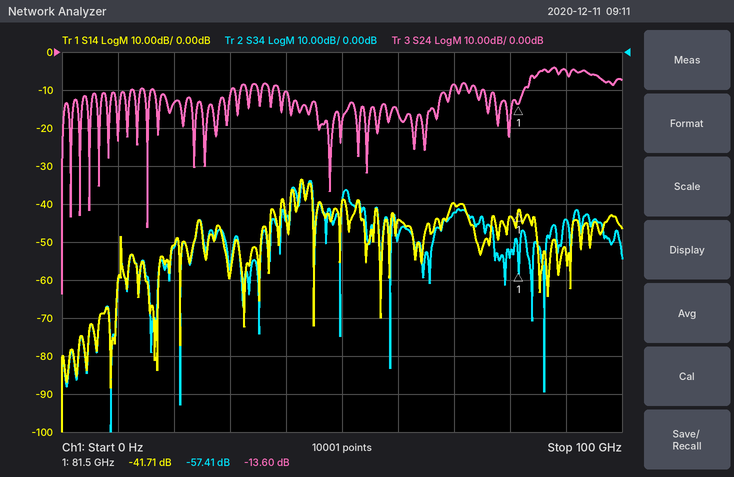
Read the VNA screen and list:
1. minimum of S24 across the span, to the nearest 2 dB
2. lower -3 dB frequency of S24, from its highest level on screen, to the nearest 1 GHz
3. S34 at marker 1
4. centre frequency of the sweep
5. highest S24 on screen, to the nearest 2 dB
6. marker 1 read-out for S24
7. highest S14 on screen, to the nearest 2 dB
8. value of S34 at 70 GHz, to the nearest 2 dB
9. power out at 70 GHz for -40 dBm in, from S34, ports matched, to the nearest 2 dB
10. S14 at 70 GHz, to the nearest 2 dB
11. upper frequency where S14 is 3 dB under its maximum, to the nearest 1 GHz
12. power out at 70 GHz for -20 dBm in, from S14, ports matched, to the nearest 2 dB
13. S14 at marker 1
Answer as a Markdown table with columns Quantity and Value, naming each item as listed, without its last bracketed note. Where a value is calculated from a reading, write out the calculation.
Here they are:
| Quantity | Value |
|---|---|
| minimum of S24 across the span, to the nearest 2 dB | -64 dB |
| lower -3 dB frequency of S24, from its highest level on screen, to the nearest 1 GHz | 84 GHz |
| S34 at marker 1 | -57.41 dB |
| centre frequency of the sweep | 50 GHz |
| highest S24 on screen, to the nearest 2 dB | -4 dB |
| marker 1 read-out for S24 | -13.60 dB |
| highest S14 on screen, to the nearest 2 dB | -34 dB |
| value of S34 at 70 GHz, to the nearest 2 dB | -42 dB |
| power out at 70 GHz for -40 dBm in, from S34, ports matched, to the nearest 2 dB | -40 dBm + (-42 dB) = -82 dBm |
| S14 at 70 GHz, to the nearest 2 dB | -40 dB |
| upper frequency where S14 is 3 dB under its maximum, to the nearest 1 GHz | 43 GHz |
| power out at 70 GHz for -20 dBm in, from S14, ports matched, to the nearest 2 dB | -20 dBm + (-40 dB) = -60 dBm |
| S14 at marker 1 | -41.71 dB |
